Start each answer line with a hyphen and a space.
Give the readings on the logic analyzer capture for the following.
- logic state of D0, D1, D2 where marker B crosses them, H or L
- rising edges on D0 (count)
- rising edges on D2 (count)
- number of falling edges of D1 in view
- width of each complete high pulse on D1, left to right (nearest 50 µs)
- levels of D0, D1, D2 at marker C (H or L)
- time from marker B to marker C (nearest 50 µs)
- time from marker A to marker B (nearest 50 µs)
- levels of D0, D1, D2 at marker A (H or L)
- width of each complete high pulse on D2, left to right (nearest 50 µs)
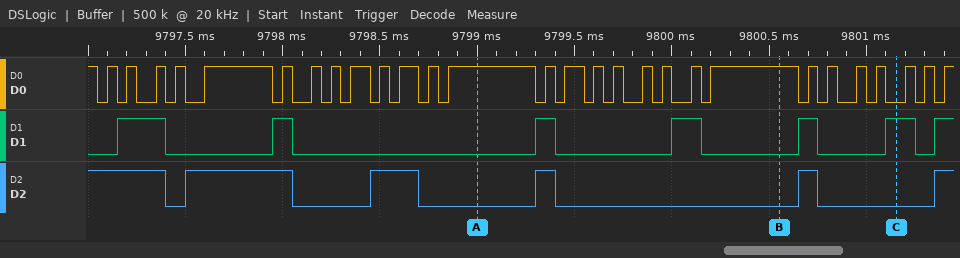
- D0=H, D1=L, D2=L
- 28
- 5
- 6
- 250 µs, 100 µs, 100 µs, 150 µs, 100 µs, 150 µs
- D0=L, D1=H, D2=L
- 600 µs
- 1550 µs
- D0=H, D1=L, D2=L
- 550 µs, 250 µs, 100 µs, 100 µs
